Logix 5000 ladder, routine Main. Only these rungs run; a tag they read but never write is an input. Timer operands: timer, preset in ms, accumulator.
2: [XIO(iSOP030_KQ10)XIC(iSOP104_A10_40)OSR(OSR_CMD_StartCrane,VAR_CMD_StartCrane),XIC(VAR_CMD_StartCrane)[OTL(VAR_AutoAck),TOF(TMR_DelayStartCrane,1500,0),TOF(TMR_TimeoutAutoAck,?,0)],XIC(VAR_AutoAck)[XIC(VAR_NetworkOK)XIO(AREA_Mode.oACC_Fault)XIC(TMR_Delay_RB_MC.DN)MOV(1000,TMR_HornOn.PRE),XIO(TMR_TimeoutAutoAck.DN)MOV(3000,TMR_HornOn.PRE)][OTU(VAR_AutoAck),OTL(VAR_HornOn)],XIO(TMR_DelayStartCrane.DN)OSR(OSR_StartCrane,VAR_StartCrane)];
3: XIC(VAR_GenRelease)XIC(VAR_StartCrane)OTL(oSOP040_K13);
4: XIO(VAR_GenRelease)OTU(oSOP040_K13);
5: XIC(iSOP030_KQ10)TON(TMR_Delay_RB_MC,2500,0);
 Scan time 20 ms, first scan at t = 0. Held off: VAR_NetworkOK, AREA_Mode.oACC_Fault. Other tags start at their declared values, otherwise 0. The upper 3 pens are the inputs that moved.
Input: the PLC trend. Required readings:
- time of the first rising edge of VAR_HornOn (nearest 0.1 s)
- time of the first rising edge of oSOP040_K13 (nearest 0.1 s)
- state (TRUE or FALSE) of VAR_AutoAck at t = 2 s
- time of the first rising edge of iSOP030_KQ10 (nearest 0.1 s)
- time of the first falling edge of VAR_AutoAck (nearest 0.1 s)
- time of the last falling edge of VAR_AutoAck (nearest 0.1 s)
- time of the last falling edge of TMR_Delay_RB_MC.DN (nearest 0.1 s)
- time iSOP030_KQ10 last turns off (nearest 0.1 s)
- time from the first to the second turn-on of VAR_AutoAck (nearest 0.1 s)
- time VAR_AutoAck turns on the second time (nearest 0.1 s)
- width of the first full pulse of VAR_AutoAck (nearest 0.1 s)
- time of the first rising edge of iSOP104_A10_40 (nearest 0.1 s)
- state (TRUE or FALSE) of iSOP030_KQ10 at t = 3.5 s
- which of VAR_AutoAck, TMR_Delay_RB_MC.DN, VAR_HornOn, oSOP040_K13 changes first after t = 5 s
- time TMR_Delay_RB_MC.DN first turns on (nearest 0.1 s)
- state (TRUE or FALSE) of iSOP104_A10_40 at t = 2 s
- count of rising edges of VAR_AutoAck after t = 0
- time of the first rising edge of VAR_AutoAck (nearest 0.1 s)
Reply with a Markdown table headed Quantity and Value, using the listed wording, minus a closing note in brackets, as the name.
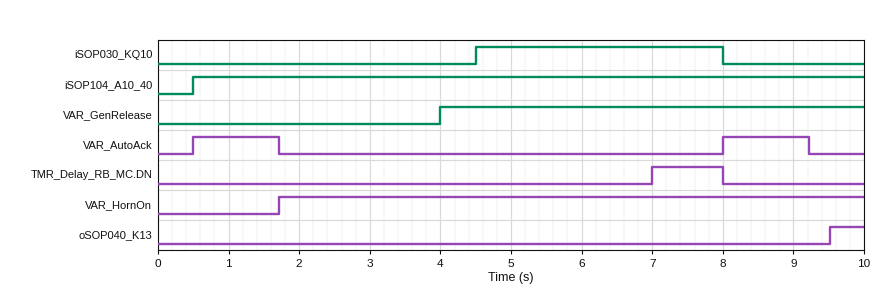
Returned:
| Quantity | Value |
|---|---|
| time of the first rising edge of VAR_HornOn | 1.7 s |
| time of the first rising edge of oSOP040_K13 | 9.5 s |
| state (TRUE or FALSE) of VAR_AutoAck at t = 2 s | FALSE |
| time of the first rising edge of iSOP030_KQ10 | 4.5 s |
| time of the first falling edge of VAR_AutoAck | 1.7 s |
| time of the last falling edge of VAR_AutoAck | 9.2 s |
| time of the last falling edge of TMR_Delay_RB_MC.DN | 8.0 s |
| time iSOP030_KQ10 last turns off | 8.0 s |
| time from the first to the second turn-on of VAR_AutoAck | 7.5 s |
| time VAR_AutoAck turns on the second time | 8.0 s |
| width of the first full pulse of VAR_AutoAck | 1.2 s |
| time of the first rising edge of iSOP104_A10_40 | 0.5 s |
| state (TRUE or FALSE) of iSOP030_KQ10 at t = 3.5 s | FALSE |
| which of VAR_AutoAck, TMR_Delay_RB_MC.DN, VAR_HornOn, oSOP040_K13 changes first after t = 5 s | TMR_Delay_RB_MC.DN |
| time TMR_Delay_RB_MC.DN first turns on | 7.0 s |
| state (TRUE or FALSE) of iSOP104_A10_40 at t = 2 s | TRUE |
| count of rising edges of VAR_AutoAck after t = 0 | 2 |
| time of the first rising edge of VAR_AutoAck | 0.5 s |
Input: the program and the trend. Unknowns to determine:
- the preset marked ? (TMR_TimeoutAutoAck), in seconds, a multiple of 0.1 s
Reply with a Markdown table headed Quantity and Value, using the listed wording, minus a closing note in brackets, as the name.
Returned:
| Quantity | Value |
|---|---|
| the preset marked ? (TMR_TimeoutAutoAck), in seconds, a multiple of 0.1 s | 1.2 s |
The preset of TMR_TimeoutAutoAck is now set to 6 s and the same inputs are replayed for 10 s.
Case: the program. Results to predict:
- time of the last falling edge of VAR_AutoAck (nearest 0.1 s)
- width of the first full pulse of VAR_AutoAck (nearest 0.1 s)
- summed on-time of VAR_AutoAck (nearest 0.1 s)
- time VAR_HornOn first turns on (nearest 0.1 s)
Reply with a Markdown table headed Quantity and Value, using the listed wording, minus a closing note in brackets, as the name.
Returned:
| Quantity | Value |
|---|---|
| time of the last falling edge of VAR_AutoAck | 6.5 s |
| width of the first full pulse of VAR_AutoAck | 6.0 s |
| summed on-time of VAR_AutoAck | 8.0 s |
| time VAR_HornOn first turns on | 6.5 s |
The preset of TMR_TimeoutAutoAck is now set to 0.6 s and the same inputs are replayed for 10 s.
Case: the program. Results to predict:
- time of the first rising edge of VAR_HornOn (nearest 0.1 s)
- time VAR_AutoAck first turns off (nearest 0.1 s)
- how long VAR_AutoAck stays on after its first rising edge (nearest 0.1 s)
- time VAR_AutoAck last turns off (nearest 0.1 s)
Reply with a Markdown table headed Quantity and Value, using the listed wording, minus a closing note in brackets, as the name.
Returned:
| Quantity | Value |
|---|---|
| time of the first rising edge of VAR_HornOn | 1.1 s |
| time VAR_AutoAck first turns off | 1.1 s |
| how long VAR_AutoAck stays on after its first rising edge | 0.6 s |
| time VAR_AutoAck last turns off | 8.6 s |
